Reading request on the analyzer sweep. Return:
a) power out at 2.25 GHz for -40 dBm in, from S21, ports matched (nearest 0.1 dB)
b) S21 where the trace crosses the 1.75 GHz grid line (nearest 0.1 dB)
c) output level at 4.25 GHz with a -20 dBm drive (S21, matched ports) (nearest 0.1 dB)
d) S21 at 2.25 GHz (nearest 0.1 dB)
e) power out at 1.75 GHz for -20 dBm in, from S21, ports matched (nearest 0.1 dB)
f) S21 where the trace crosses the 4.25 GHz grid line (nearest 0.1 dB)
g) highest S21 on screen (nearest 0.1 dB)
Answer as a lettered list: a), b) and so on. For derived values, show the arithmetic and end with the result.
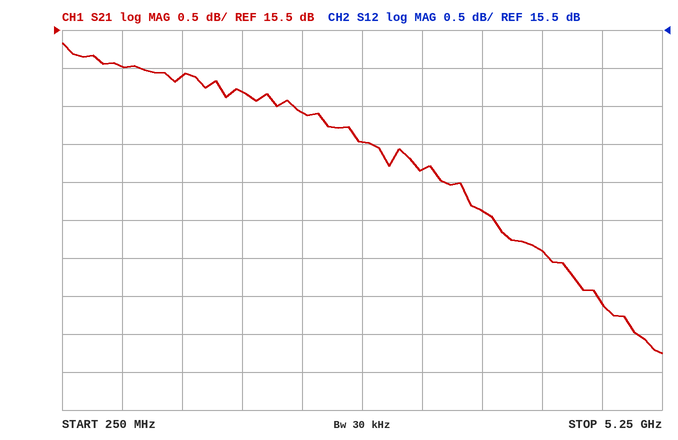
a) -40 dBm + (14.4 dB) = -25.6 dBm
b) 14.7 dB
c) -20 dBm + (12.6 dB) = -7.4 dBm
d) 14.4 dB
e) -20 dBm + (14.7 dB) = -5.3 dBm
f) 12.6 dB
g) 15.3 dB
